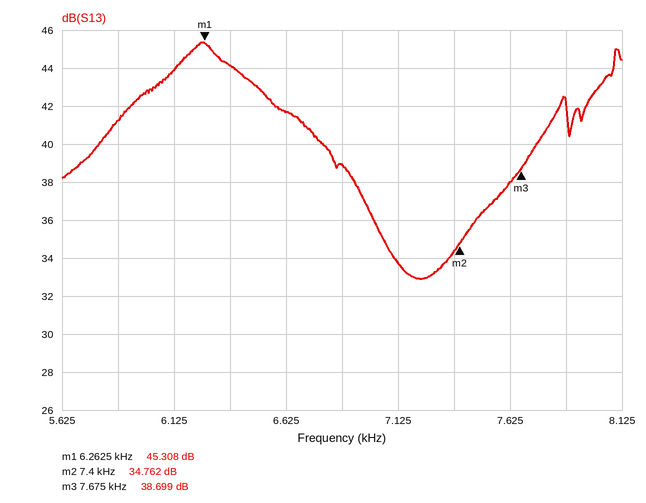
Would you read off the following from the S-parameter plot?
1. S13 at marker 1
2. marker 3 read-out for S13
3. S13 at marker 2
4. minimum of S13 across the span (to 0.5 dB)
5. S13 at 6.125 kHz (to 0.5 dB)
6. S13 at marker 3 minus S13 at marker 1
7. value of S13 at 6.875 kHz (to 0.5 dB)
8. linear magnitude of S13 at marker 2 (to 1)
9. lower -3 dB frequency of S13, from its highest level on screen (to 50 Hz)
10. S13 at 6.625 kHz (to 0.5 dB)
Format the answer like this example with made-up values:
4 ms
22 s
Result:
45.308 dB
38.699 dB
34.762 dB
33.0 dB
44.0 dB
-6.609 dB
39.0 dB
55
5.95 kHz
41.5 dB
